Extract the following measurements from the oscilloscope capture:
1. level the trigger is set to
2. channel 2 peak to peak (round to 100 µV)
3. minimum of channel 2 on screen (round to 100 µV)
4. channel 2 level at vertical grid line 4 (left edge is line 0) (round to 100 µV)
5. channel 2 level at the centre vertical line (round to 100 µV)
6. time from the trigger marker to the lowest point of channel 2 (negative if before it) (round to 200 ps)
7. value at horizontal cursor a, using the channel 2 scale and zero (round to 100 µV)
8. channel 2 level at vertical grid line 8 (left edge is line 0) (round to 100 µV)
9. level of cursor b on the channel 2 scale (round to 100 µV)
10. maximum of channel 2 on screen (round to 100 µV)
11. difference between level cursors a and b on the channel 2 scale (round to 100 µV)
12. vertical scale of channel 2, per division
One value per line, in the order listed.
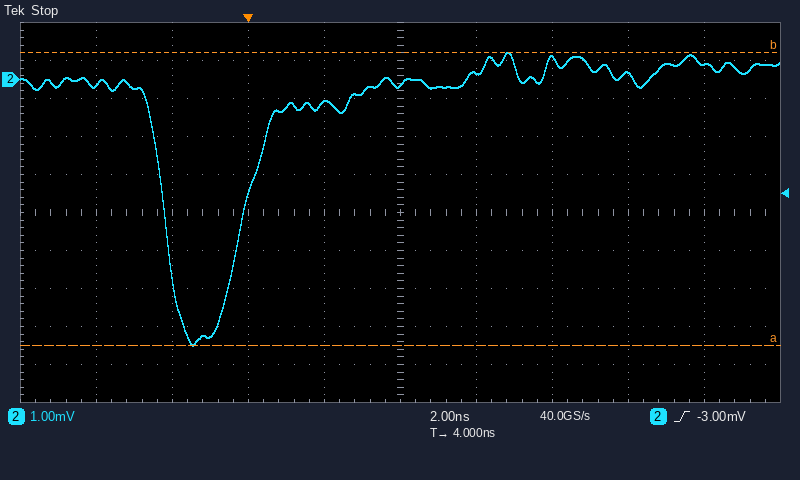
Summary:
-3.00 mV
7.7 mV
-7.0 mV
-600 µV
-100 µV
-1.4 ns
-7.0 mV
100 µV
700 µV
700 µV
7.7 mV
1 mV
